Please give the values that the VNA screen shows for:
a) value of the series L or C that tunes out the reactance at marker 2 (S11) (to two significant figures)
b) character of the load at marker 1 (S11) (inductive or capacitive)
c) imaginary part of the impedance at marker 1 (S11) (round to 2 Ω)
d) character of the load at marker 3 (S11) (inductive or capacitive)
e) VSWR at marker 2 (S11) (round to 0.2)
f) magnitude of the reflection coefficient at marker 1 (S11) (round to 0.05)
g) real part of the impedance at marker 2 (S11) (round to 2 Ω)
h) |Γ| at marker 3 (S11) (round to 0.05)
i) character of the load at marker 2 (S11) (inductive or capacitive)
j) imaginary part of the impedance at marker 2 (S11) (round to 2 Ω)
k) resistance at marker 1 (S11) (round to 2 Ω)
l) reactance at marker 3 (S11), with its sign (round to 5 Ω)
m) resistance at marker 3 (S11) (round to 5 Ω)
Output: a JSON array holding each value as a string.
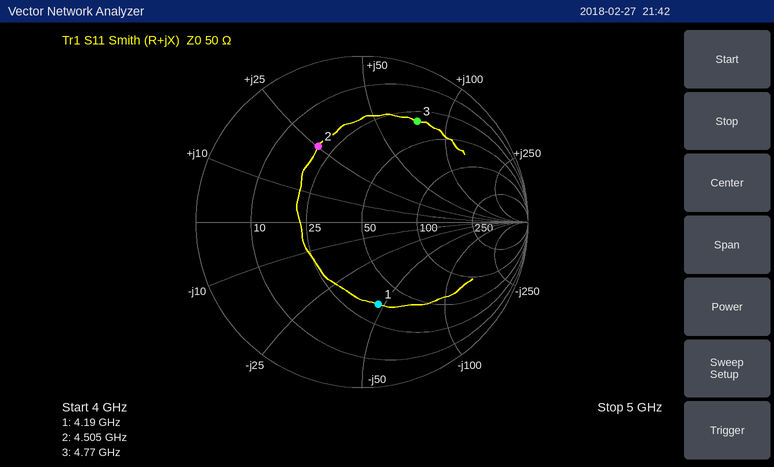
["1.4 pF", "capacitive", "-46 Ω", "inductive", "3.2", "0.50", "20 Ω", "0.70", "inductive", "+26 Ω", "36 Ω", "+75 Ω", "30 Ω"]
